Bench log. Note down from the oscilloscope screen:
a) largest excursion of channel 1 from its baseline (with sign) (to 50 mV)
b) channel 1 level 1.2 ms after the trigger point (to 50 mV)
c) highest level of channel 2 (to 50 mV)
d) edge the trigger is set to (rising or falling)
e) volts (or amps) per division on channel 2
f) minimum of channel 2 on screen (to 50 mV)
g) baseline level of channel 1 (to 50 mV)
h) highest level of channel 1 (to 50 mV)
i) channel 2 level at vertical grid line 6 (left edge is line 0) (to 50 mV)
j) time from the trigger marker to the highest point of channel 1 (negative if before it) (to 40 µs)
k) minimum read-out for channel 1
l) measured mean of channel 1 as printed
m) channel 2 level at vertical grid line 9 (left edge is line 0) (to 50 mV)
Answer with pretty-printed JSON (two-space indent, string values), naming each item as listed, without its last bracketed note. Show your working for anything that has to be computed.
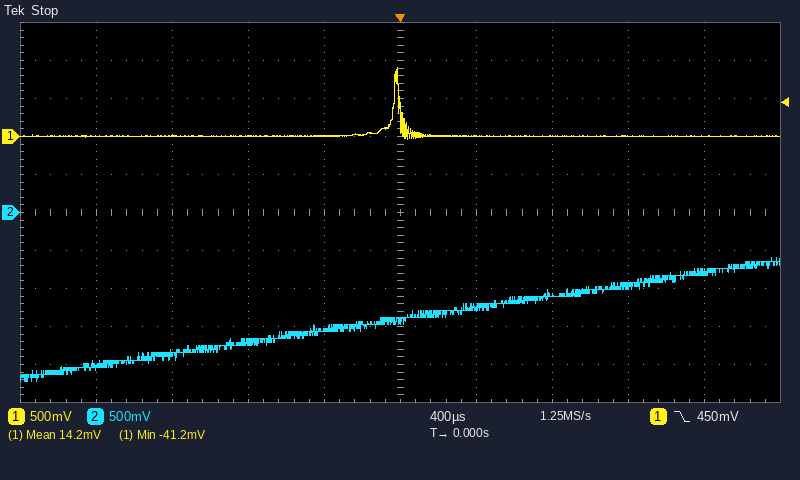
{
  "largest excursion of channel 1 from its baseline (with sign)": "900 mV − (0 mV) = +900 mV",
  "channel 1 level 1.2 ms after the trigger point": "0 mV",
  "highest level of channel 2": "-600 mV",
  "edge the trigger is set to": "falling",
  "volts (or amps) per division on channel 2": "500 mV",
  "minimum of channel 2 on screen": "-2.20 V",
  "baseline level of channel 1": "0 mV",
  "highest level of channel 1": "900 mV",
  "channel 2 level at vertical grid line 6 (left edge is line 0)": "-1.25 V",
  "time from the trigger marker to the highest point of channel 1 (negative if before it)": "0 µs",
  "minimum read-out for channel 1": "-41.2 mV",
  "measured mean of channel 1 as printed": "14.2 mV",
  "channel 2 level at vertical grid line 9 (left edge is line 0)": "-800 mV"
}
